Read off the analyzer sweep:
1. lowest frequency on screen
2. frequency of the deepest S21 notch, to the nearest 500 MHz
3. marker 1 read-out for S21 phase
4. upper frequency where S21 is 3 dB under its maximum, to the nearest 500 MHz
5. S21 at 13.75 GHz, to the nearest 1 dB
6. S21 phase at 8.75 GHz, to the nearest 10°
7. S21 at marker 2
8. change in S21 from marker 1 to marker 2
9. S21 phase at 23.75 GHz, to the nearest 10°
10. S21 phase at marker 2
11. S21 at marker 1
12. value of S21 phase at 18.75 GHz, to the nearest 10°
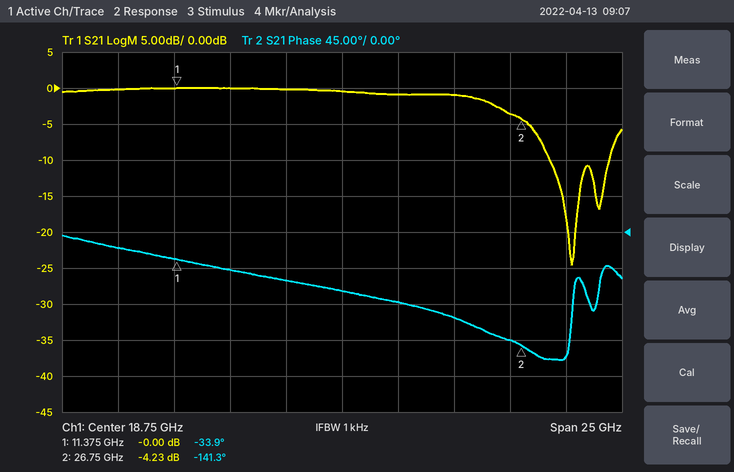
6.25 GHz
29.0 GHz
-33.9°
26.0 GHz
0 dB
-20°
-4.23 dB
-4.23 dB
-110°
-141.3°
-0.00 dB
-70°
